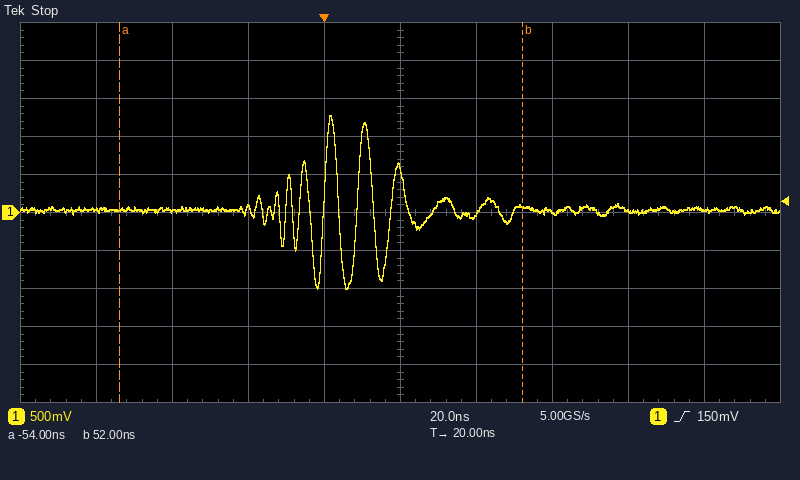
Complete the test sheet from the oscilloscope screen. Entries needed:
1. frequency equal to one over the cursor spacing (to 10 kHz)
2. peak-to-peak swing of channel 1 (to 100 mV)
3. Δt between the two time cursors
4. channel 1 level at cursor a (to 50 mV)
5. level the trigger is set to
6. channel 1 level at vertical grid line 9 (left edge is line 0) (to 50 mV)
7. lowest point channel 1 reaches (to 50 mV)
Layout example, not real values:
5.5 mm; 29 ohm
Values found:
9.43 MHz; 2.30 V; 106 ns; 50 mV; 150 mV; 50 mV; -1.00 V
